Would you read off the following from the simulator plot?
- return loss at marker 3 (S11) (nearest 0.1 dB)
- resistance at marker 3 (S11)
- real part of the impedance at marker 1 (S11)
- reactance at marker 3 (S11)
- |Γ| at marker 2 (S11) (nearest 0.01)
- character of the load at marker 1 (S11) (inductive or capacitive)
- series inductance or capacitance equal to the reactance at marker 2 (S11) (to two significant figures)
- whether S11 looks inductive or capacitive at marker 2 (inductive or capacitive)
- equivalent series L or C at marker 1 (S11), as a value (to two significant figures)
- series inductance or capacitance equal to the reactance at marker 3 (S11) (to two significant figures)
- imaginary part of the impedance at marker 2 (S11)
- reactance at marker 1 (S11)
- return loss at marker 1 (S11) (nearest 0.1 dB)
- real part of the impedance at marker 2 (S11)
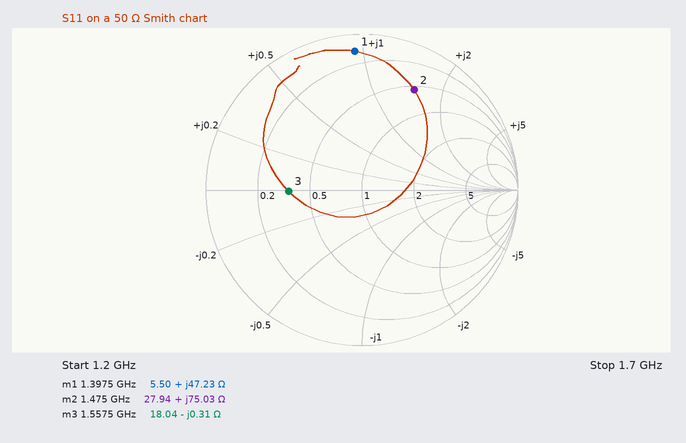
6.6 dB
18.04 Ω
5.50 Ω
-0.31 Ω
0.72
inductive
8.1 nH
inductive
5.4 nH
330 pF
+75.03 Ω
+47.23 Ω
1.0 dB
27.94 Ω
